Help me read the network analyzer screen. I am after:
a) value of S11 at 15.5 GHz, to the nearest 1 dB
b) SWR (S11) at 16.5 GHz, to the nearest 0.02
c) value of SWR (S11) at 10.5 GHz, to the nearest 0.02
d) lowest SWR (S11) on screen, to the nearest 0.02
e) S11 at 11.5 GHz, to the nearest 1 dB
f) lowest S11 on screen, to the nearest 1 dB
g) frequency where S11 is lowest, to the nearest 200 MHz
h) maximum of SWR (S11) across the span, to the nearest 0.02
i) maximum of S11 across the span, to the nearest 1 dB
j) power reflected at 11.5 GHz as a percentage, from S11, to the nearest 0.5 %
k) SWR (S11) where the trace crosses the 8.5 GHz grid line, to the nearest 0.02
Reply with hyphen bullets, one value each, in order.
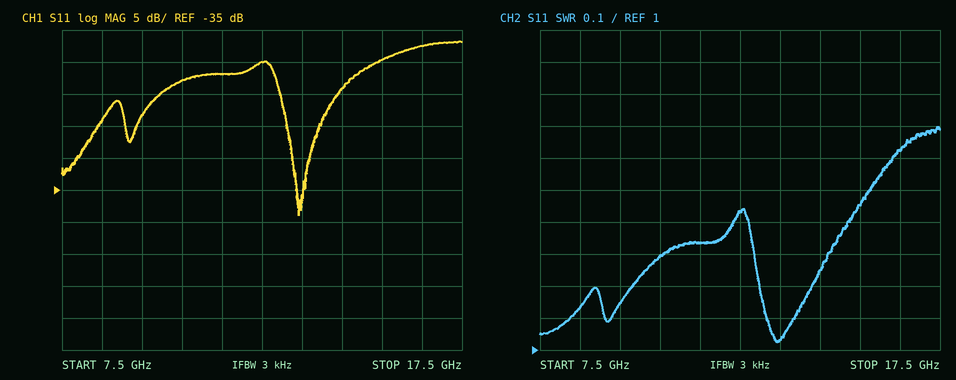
- -15 dB
- 1.62
- 1.30
- 1.02
- -17 dB
- -39 dB
- 13.4 GHz
- 1.70
- -12 dB
- 2.0 %
- 1.14
